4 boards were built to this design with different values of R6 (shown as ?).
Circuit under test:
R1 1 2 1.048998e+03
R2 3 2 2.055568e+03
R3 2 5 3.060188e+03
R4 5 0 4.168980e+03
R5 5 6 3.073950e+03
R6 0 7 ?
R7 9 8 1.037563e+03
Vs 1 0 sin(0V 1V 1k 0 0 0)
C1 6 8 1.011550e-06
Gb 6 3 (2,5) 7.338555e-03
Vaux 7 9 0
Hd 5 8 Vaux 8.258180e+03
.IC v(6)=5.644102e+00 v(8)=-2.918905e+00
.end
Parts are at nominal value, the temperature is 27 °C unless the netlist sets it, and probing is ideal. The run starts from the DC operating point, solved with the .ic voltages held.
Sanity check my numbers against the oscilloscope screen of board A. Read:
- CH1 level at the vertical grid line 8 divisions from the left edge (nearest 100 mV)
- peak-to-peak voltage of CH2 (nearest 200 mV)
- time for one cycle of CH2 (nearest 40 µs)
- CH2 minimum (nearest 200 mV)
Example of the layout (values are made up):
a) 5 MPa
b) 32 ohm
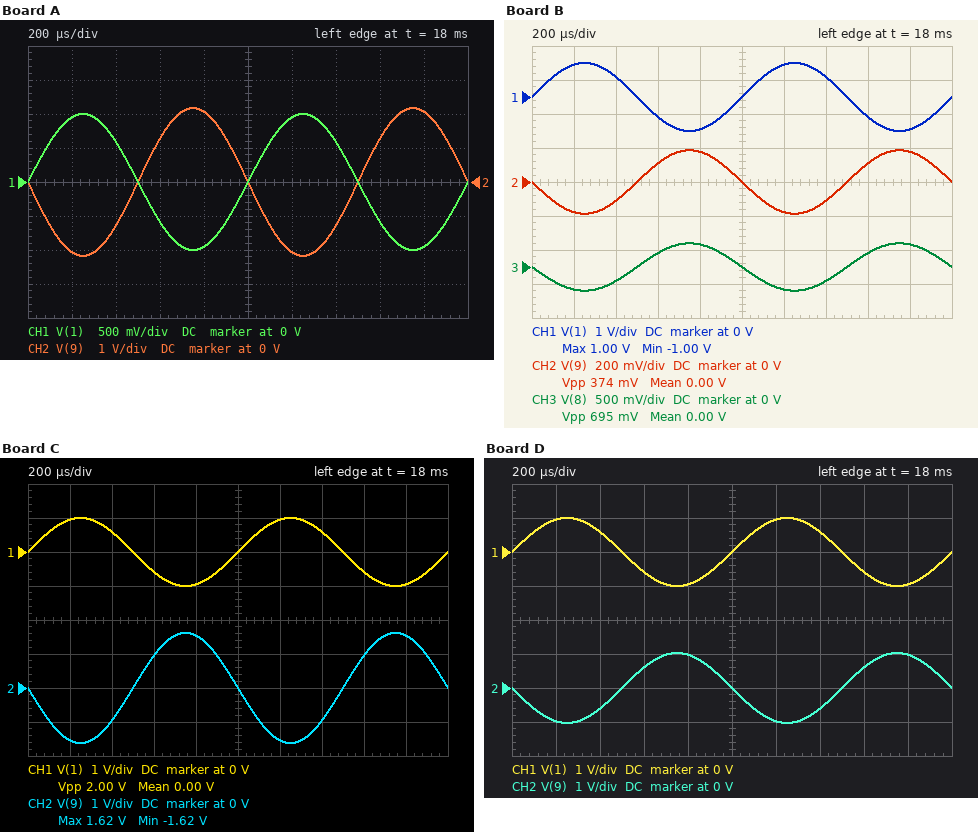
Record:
a) -600 mV
b) 4.4 V
c) 1.00 ms
d) -2.2 V
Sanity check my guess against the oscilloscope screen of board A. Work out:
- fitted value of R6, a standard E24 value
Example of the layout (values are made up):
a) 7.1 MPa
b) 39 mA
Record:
a) 4.7 kΩ
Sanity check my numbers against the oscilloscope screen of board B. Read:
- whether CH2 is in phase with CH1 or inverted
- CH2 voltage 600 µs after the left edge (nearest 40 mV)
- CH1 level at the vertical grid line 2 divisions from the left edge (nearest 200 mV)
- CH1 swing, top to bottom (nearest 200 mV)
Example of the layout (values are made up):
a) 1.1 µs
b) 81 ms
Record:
a) inverted
b) 120 mV
c) 600 mV
d) 2.0 V
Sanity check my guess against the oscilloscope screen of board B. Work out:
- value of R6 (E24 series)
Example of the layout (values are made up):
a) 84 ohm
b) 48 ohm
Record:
a) 1.2 kΩ
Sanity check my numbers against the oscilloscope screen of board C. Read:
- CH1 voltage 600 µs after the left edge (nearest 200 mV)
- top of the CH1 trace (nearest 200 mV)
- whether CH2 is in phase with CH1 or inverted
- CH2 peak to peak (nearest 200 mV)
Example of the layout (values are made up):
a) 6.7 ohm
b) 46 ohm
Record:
a) -600 mV
b) 1.0 V
c) inverted
d) 3.2 V
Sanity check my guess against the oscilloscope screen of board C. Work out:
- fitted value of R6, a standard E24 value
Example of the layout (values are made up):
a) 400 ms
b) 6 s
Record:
a) 4.3 kΩ
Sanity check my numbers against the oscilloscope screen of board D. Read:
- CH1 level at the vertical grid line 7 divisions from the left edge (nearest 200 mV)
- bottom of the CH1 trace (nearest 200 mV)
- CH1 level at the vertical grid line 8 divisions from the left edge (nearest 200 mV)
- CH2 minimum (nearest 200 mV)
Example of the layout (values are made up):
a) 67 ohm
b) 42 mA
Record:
a) 600 mV
b) -1.0 V
c) -600 mV
d) -1.0 V
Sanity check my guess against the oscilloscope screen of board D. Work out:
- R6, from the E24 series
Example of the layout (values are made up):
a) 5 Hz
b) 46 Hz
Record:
a) 3.6 kΩ
